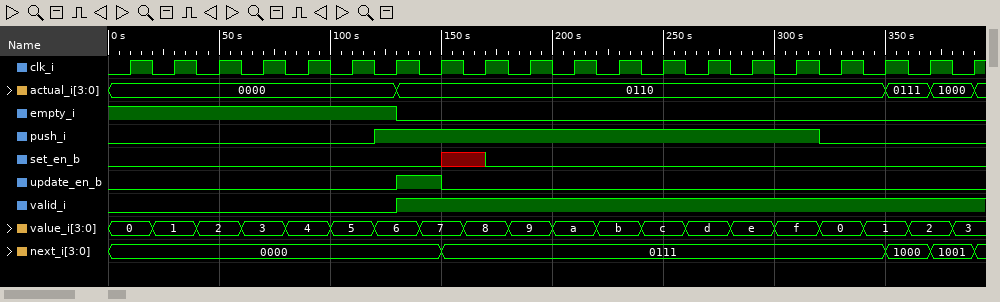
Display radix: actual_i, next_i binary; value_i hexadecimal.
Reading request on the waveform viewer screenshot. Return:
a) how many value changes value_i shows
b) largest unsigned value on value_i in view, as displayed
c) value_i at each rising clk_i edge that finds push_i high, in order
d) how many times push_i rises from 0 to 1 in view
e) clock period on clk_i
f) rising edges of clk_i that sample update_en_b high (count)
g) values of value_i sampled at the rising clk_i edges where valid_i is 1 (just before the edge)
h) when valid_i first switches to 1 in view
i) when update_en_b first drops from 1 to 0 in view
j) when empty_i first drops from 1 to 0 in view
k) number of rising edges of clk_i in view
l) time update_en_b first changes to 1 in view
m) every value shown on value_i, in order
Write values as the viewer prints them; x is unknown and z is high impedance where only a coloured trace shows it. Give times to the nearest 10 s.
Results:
19
f
6, 7, 8, 9, a, b, c, d, e, f
1
20 s
1
7, 8, 9, a, b, c, d, e, f, 0, 1, 2, 3
130 s
150 s
130 s
20
130 s
0, 1, 2, 3, 4, 5, 6, 7, 8, 9, a, b, c, d, e, f, 0, 1, 2, 3
